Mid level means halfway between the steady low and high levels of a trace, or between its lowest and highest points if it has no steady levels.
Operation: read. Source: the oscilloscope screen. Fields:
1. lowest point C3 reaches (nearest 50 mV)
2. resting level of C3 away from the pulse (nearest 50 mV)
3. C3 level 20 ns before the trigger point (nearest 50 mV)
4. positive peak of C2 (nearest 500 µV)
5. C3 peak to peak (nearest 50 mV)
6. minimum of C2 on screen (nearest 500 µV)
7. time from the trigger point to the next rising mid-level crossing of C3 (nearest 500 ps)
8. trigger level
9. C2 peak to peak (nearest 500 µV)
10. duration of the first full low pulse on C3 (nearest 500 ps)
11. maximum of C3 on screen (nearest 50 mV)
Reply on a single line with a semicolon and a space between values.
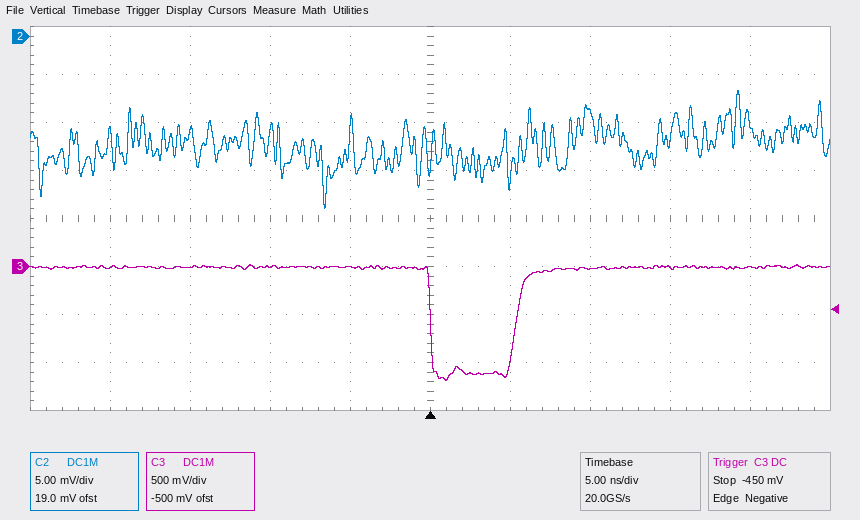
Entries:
-1.20 V; 0 mV; 0 mV; -5.5 mV; 1.20 V; -18.0 mV; 5.5 ns; -450 mV; 12.5 mV; 5.5 ns; 0 mV
